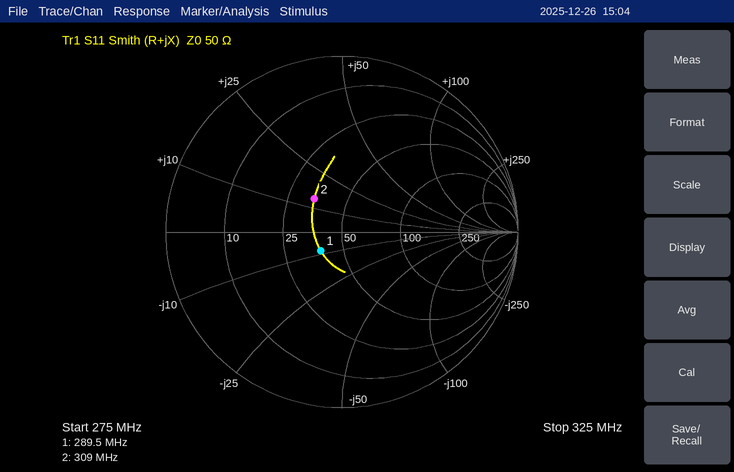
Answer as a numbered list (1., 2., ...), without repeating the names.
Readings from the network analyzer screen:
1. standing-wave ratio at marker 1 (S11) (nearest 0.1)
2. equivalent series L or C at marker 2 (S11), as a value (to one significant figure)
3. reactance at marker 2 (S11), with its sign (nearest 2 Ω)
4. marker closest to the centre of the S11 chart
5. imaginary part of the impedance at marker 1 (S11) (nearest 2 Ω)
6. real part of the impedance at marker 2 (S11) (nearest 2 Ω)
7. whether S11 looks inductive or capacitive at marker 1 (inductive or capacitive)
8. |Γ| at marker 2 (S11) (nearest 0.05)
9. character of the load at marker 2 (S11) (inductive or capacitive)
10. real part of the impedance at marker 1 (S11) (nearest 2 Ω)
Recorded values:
1. 1.4
2. 7 nH
3. +14 Ω
4. marker 1
5. -8 Ω
6. 34 Ω
7. capacitive
8. 0.25
9. inductive
10. 38 Ω
